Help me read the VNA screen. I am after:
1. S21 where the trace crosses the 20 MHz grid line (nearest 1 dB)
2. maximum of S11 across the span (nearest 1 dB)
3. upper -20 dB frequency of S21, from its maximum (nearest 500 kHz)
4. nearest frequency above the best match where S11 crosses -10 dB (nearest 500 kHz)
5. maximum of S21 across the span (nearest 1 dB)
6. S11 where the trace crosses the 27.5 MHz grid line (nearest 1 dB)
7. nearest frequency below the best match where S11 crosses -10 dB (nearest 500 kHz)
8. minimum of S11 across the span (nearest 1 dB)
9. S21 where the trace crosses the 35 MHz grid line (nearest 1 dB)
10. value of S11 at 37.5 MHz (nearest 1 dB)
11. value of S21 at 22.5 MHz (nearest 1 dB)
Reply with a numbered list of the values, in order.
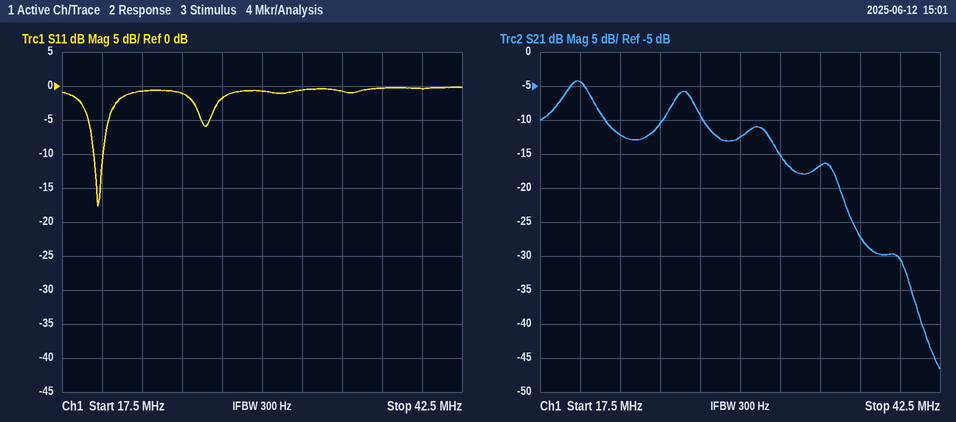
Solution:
1. -4 dB
2. 0 dB
3. 37.0 MHz
4. 20.0 MHz
5. -4 dB
6. -2 dB
7. 19.5 MHz
8. -18 dB
9. -17 dB
10. 0 dB
11. -12 dB
